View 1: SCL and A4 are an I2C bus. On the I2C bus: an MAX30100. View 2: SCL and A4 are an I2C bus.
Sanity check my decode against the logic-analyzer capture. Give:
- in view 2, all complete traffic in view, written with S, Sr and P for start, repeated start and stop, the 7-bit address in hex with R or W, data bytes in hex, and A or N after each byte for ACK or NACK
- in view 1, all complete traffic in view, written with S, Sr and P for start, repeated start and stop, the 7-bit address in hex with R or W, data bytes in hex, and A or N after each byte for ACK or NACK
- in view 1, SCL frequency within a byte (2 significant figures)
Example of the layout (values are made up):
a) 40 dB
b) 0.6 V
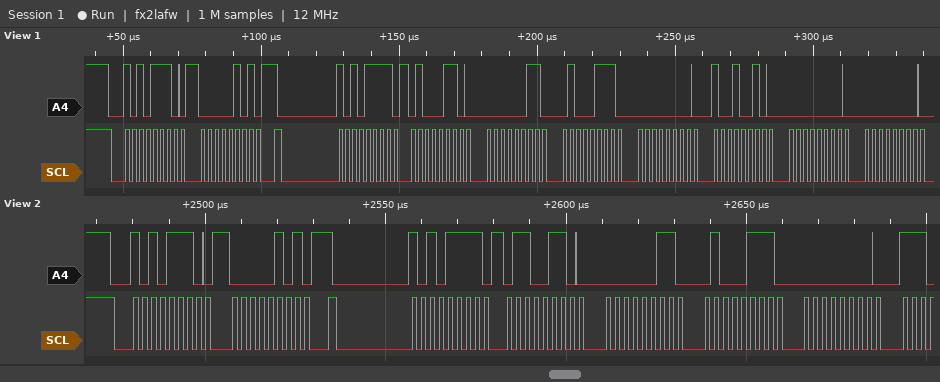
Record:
a) S 57W A 05 A Sr 57R A 66 A 03 A 47 A 00 A
b) S 57W A 05 A Sr 57R A 46 A 03 A 47 A 00 A 92 A 00 A 00 A
c) 400 kHz
